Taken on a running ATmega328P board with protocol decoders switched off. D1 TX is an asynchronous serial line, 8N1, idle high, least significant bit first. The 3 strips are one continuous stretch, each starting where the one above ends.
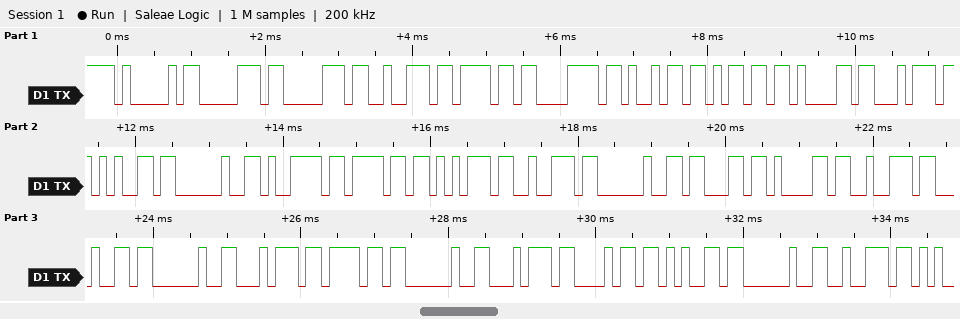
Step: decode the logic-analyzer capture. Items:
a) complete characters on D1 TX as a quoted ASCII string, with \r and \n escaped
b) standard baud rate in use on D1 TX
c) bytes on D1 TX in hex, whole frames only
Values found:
"Approximate your card to the r"
9600 baud
41 70 70 72 6F 78 69 6D 61 74 65 20 79 6F 75 72 20 63 61 72 64 20 74 6F 20 74 68 65 20 72
